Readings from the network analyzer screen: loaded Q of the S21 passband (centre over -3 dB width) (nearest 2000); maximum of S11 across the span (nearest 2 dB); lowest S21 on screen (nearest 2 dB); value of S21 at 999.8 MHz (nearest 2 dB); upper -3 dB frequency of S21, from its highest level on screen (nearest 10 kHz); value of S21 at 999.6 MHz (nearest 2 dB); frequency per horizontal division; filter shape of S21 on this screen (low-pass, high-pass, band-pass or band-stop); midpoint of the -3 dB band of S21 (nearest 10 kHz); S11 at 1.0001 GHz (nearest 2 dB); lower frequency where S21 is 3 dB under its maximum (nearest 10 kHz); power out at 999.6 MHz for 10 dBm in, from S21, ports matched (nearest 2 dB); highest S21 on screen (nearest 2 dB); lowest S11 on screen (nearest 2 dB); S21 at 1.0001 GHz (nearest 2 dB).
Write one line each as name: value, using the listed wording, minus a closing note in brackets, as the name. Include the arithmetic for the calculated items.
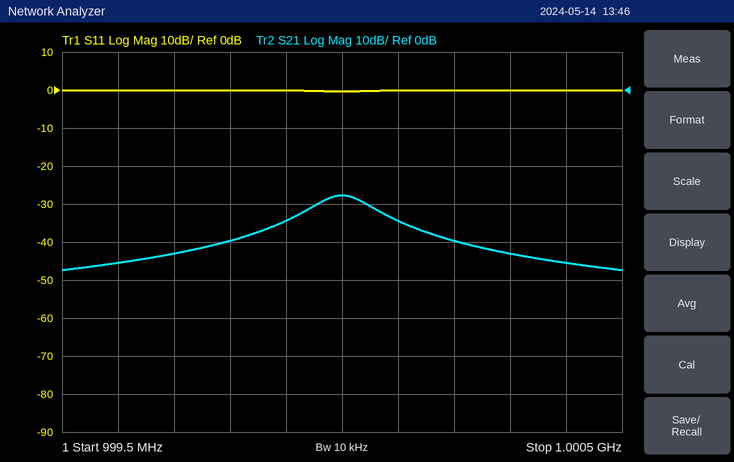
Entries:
loaded Q of the S21 passband (centre over -3 dB width): 1 GHz / 100 kHz ≈ 10000
maximum of S11 across the span: 0 dB
lowest S21 on screen: -48 dB
value of S21 at 999.8 MHz: -40 dB
upper -3 dB frequency of S21, from its highest level on screen: 1.00005 GHz
value of S21 at 999.6 MHz: -46 dB
frequency per horizontal division: 100 kHz
filter shape of S21 on this screen: band-pass
midpoint of the -3 dB band of S21: 1.00000 GHz
S11 at 1.0001 GHz: 0 dB
lower frequency where S21 is 3 dB under its maximum: 999.95 MHz
power out at 999.6 MHz for 10 dBm in, from S21, ports matched: 10 dBm + (-46 dB) = -36 dBm
highest S21 on screen: -28 dB
lowest S11 on screen: 0 dB
S21 at 1.0001 GHz: -34 dB
